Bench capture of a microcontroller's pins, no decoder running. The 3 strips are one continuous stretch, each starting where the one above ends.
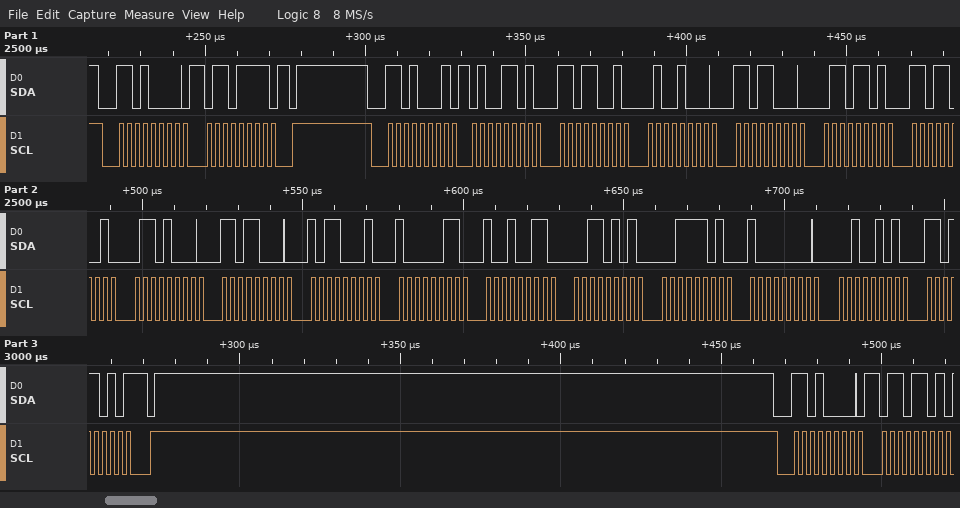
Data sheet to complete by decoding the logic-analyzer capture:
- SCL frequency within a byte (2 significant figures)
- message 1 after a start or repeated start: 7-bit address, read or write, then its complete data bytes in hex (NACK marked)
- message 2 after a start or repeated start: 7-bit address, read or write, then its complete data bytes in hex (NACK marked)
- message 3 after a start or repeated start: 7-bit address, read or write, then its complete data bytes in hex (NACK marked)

400 kHz
0x68 write: 6F
0x68 read: 4D D9 48 D8 6D D9 68 D8 B1 83 93 35 3D 80 25 DA NACK
0x68 write: 6D
